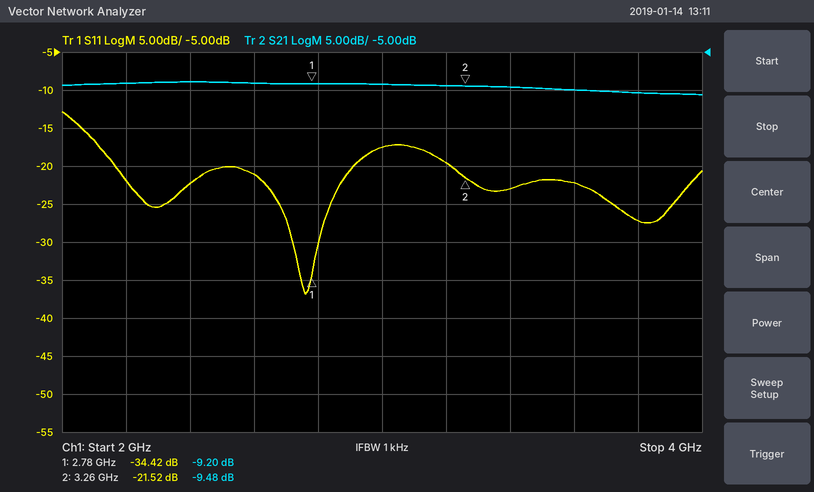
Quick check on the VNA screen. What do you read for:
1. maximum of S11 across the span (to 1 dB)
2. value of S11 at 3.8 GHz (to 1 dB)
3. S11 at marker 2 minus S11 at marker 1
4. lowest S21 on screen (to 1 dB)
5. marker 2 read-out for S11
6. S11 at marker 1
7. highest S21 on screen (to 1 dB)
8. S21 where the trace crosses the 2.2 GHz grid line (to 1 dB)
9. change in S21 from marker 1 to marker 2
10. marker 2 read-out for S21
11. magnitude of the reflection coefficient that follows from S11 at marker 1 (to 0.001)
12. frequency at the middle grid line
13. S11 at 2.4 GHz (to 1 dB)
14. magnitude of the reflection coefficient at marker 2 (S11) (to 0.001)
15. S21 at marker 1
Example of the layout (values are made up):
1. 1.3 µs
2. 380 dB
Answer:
1. -13 dB
2. -27 dB
3. 12.90 dB
4. -11 dB
5. -21.52 dB
6. -34.42 dB
7. -9 dB
8. -9 dB
9. -0.28 dB
10. -9.48 dB
11. 0.019
12. 3 GHz
13. -22 dB
14. 0.084
15. -9.20 dB
